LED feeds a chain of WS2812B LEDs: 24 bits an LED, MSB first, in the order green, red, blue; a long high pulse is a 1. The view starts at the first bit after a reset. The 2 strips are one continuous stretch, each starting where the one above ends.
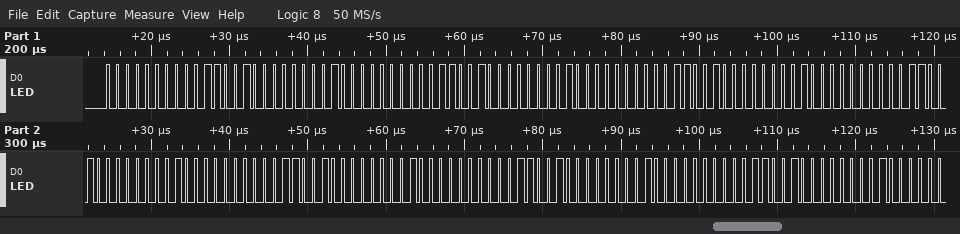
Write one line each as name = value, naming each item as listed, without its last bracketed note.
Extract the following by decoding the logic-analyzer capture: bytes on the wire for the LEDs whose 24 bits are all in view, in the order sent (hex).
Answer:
bytes on the wire for the LEDs whose 24 bits are all in view, in the order sent = 00 32 01 00 32 01 00 32 01 00 32 01 00 32 01 00 32 01 00 32 01
